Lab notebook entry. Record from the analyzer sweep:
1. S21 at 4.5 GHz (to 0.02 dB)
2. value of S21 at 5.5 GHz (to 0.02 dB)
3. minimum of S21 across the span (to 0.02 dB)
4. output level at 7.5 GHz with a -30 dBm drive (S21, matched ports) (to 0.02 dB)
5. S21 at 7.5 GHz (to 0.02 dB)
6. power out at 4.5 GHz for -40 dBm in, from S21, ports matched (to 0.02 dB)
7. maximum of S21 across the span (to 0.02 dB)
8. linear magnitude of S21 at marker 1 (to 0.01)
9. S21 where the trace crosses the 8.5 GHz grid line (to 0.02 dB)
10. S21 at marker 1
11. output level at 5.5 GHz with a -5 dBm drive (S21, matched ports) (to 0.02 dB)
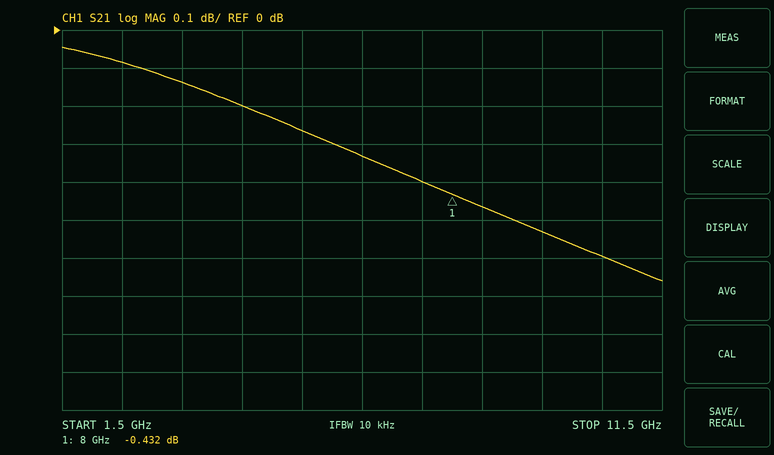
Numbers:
-0.20 dB
-0.26 dB
-0.66 dB
-30.40 dBm
-0.40 dB
-40.20 dBm
-0.04 dB
0.95
-0.46 dB
-0.432 dB
-5.26 dBm
